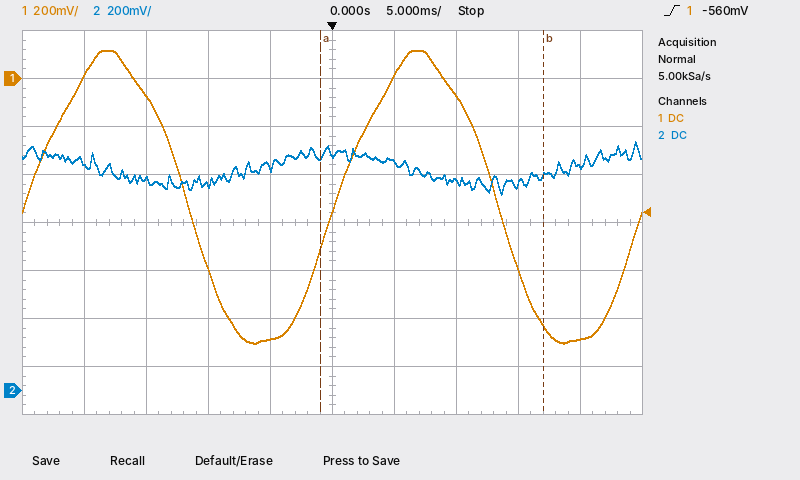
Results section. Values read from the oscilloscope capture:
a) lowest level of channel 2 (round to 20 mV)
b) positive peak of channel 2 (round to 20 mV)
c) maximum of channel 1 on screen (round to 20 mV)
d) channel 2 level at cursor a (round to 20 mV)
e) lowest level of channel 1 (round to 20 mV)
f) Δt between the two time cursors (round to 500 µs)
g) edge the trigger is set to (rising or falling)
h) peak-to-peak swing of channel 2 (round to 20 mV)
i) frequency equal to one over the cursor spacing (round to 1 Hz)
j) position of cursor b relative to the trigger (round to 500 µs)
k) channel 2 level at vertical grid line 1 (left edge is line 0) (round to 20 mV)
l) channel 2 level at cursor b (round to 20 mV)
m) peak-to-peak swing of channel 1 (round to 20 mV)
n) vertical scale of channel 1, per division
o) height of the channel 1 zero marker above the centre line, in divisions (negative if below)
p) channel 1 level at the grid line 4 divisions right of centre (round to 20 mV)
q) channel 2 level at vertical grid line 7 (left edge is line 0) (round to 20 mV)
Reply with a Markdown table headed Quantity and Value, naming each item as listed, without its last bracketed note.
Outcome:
| Quantity | Value |
|---|---|
| lowest level of channel 2 | 820 mV |
| positive peak of channel 2 | 1.04 V |
| maximum of channel 1 on screen | 120 mV |
| channel 2 level at cursor a | 980 mV |
| lowest level of channel 1 | -1.10 V |
| Δt between the two time cursors | 18.0 ms |
| edge the trigger is set to | rising |
| peak-to-peak swing of channel 2 | 220 mV |
| frequency equal to one over the cursor spacing | 56 Hz |
| position of cursor b relative to the trigger | +17.0 ms |
| channel 2 level at vertical grid line 1 (left edge is line 0) | 940 mV |
| channel 2 level at cursor b | 900 mV |
| peak-to-peak swing of channel 1 | 1.22 V |
| vertical scale of channel 1, per division | 200 mV |
| height of the channel 1 zero marker above the centre line, in divisions | +3.0 div |
| channel 1 level at the grid line 4 divisions right of centre | -1.08 V |
| channel 2 level at vertical grid line 7 (left edge is line 0) | 880 mV |
